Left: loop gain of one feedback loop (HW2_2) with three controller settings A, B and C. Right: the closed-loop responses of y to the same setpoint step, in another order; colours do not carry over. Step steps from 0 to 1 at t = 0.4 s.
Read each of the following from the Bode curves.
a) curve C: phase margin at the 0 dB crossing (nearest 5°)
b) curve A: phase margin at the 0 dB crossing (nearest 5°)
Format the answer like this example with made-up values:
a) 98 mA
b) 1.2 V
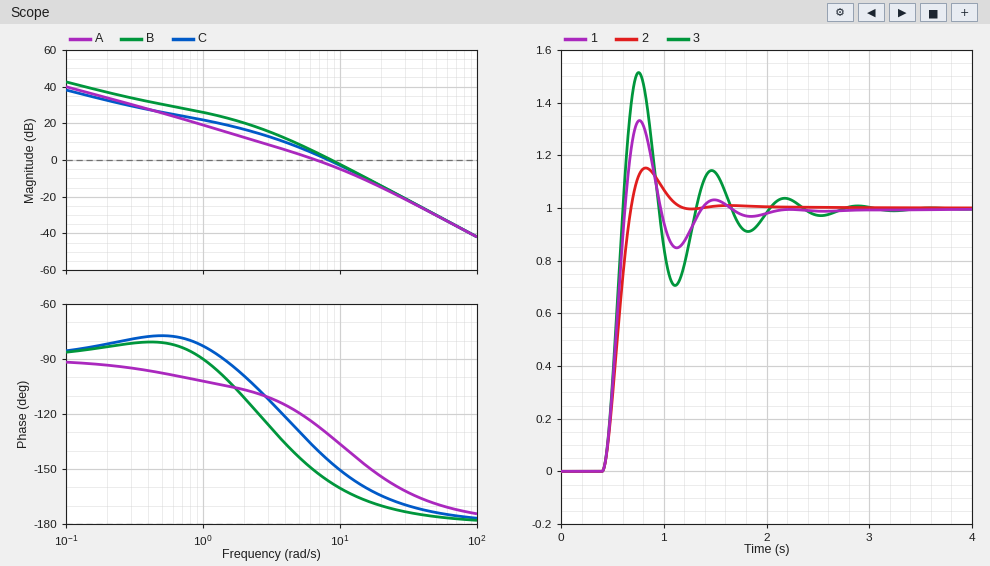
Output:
a) 35°
b) 55°
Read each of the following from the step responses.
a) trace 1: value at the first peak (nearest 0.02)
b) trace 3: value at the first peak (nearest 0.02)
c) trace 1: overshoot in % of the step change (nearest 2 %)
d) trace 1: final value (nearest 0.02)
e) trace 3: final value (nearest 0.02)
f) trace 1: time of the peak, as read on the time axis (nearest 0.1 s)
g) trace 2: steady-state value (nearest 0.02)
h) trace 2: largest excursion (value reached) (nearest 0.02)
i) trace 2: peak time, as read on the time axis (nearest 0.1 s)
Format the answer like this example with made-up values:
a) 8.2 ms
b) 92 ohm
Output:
a) 1.34
b) 1.52
c) 34 %
d) 1.00
e) 1.00
f) 0.8 s
g) 1.00
h) 1.16
i) 0.8 s
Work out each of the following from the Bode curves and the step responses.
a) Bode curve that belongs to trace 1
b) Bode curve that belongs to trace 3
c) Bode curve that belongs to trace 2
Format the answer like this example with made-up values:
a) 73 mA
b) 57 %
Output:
a) C
b) B
c) A
